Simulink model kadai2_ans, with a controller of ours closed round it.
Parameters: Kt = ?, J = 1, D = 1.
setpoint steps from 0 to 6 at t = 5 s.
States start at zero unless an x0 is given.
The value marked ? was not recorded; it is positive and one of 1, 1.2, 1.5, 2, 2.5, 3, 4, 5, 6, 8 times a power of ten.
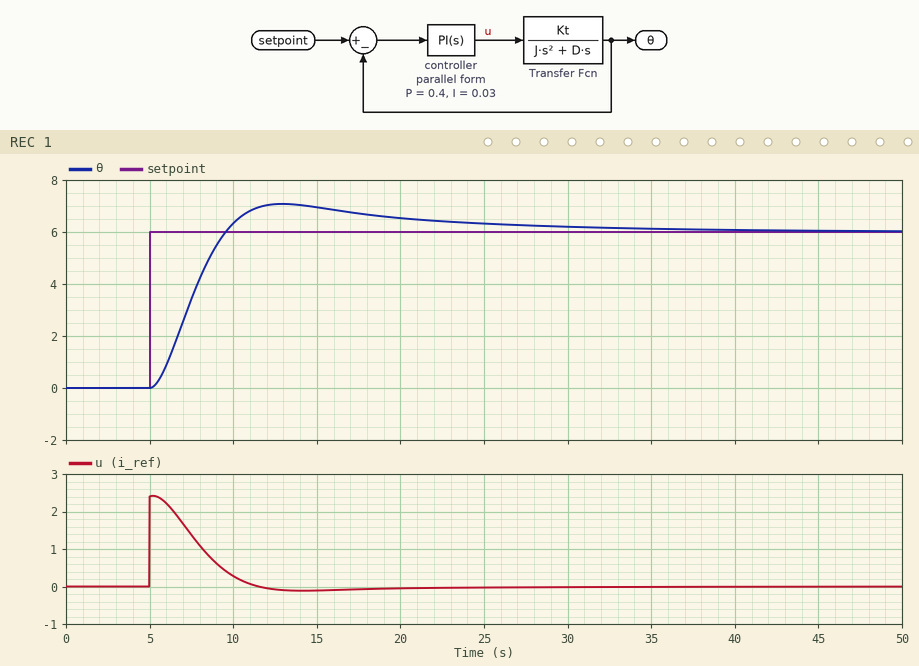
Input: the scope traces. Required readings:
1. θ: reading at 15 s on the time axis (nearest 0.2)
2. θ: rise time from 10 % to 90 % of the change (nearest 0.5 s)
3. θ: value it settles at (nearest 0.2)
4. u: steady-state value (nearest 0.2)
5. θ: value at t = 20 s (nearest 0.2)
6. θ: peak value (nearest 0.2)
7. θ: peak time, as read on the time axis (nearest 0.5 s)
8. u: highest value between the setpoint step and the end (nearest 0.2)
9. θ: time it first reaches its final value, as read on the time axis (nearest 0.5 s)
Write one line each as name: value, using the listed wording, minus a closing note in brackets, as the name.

θ: reading at 15 s on the time axis: 7.0
θ: rise time from 10 % to 90 % of the change: 3.0 s
θ: value it settles at: 6.0
u: steady-state value: 0.0
θ: value at t = 20 s: 6.6
θ: peak value: 7.0
θ: peak time, as read on the time axis: 13.0 s
u: highest value between the setpoint step and the end: 2.4
θ: time it first reaches its final value, as read on the time axis: 9.5 s
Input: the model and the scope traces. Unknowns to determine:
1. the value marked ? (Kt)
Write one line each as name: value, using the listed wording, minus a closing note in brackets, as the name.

the value marked ?: 1
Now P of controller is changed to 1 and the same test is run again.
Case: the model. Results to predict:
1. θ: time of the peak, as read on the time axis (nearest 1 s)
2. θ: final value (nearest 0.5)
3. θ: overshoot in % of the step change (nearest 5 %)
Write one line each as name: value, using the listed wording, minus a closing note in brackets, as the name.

θ: time of the peak, as read on the time axis: 9 s
θ: final value: 6.0
θ: overshoot in % of the step change: 20 %
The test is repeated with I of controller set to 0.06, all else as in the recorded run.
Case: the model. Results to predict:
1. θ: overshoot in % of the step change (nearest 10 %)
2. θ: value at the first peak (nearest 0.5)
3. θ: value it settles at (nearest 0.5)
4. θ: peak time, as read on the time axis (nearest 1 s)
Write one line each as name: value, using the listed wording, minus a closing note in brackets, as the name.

θ: overshoot in % of the step change: 30 %
θ: value at the first peak: 8.0
θ: value it settles at: 6.0
θ: peak time, as read on the time axis: 12 s
